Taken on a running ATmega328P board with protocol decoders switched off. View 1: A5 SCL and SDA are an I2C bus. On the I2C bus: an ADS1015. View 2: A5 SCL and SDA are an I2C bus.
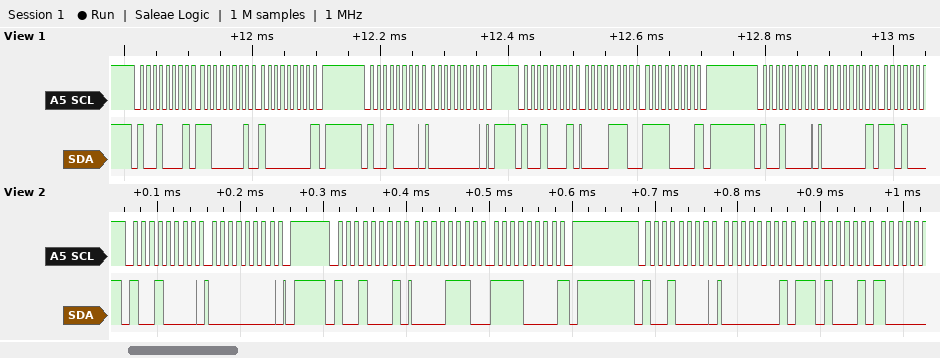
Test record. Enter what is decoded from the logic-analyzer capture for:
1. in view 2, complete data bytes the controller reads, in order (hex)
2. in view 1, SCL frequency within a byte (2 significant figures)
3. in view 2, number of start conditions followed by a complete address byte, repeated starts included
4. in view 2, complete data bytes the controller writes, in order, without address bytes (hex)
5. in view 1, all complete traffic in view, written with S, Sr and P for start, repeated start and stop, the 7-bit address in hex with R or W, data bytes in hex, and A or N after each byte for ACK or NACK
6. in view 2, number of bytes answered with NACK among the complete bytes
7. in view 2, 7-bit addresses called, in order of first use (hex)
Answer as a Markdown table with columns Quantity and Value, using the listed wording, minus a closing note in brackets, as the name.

| Quantity | Value |
|---|---|
| in view 2, complete data bytes the controller reads, in order | 0E F0 |
| in view 1, SCL frequency within a byte | 100 kHz |
| in view 2, number of start conditions followed by a complete address byte, repeated starts included | 3 |
| in view 2, complete data bytes the controller writes, in order, without address bytes | 00 01 D1 |
| in view 1, all complete traffic in view, written with S, Sr and P for start, repeated start and stop, the 7-bit address in hex with R or W, data bytes in hex, and A or N after each byte for ACK or NACK | S 48R A C1 A 80 N P S 48W A 00 A P S 48R A 0E A F0 N P S 48W A 01 A |
| in view 2, number of bytes answered with NACK among the complete bytes | 1 |
| in view 2, 7-bit addresses called, in order of first use | 0x48 |
